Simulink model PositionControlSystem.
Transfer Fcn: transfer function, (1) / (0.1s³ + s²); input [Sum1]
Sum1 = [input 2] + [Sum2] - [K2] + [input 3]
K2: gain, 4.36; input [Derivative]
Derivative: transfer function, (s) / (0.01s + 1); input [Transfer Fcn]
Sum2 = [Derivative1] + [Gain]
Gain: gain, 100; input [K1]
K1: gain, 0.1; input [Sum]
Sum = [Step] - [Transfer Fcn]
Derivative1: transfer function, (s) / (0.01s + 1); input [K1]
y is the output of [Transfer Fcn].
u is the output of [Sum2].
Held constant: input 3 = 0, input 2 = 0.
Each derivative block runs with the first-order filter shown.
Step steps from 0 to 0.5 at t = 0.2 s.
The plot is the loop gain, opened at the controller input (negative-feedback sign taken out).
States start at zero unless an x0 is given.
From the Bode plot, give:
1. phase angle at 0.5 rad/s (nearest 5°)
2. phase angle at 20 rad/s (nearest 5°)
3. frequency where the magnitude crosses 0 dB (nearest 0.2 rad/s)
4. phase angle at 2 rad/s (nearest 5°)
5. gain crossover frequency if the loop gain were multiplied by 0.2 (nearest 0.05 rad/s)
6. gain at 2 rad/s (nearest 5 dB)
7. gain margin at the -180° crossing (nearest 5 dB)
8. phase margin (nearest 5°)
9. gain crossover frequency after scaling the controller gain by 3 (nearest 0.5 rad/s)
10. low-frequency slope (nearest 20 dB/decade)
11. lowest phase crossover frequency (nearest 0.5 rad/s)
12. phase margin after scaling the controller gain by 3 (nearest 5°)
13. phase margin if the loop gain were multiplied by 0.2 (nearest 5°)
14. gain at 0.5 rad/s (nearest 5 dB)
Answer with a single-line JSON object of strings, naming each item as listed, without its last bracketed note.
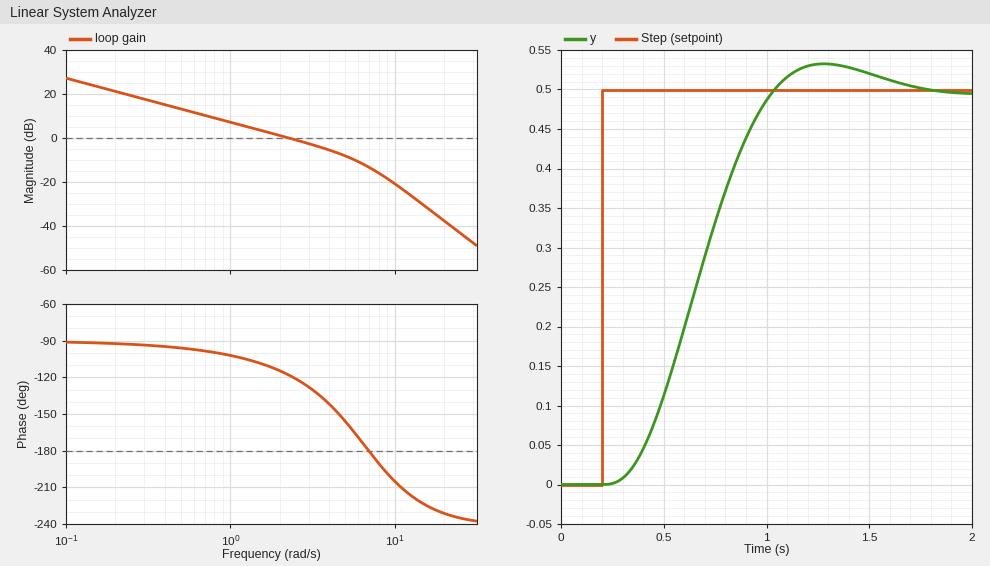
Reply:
{"phase angle at 0.5 rad/s": "-95°", "phase angle at 20 rad/s": "-230°", "frequency where the magnitude crosses 0 dB": "2.2 rad/s", "phase angle at 2 rad/s": "-115°", "gain crossover frequency if the loop gain were multiplied by 0.2": "0.45 rad/s", "gain at 2 rad/s": "0 dB", "gain margin at the -180° crossing": "15 dB", "phase margin": "60°", "gain crossover frequency after scaling the controller gain by 3": "5.5 rad/s", "low-frequency slope": "-20 dB/decade", "lowest phase crossover frequency": "7.0 rad/s", "phase margin after scaling the controller gain by 3": "15°", "phase margin if the loop gain were multiplied by 0.2": "85°", "gain at 0.5 rad/s": "15 dB"}
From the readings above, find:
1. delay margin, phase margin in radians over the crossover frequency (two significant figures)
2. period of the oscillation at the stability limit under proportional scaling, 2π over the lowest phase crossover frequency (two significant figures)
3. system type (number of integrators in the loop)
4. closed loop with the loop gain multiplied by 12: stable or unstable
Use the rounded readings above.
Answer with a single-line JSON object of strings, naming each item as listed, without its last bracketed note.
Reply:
{"delay margin, phase margin in radians over the crossover frequency": "0.48 s", "period of the oscillation at the stability limit under proportional scaling, 2π over the lowest phase crossover frequency": "0.90 s", "system type": "1", "closed loop with the loop gain multiplied by 12: stable or unstable": "unstable"}
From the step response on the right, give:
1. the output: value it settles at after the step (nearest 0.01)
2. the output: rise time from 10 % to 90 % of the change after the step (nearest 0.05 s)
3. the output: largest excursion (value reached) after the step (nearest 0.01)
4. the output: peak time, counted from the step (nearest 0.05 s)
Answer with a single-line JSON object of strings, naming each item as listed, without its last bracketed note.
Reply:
{"the output: value it settles at after the step": "0.50", "the output: rise time from 10 % to 90 % of the change after the step": "0.50 s", "the output: largest excursion (value reached) after the step": "0.53", "the output: peak time, counted from the step": "1.10 s"}
